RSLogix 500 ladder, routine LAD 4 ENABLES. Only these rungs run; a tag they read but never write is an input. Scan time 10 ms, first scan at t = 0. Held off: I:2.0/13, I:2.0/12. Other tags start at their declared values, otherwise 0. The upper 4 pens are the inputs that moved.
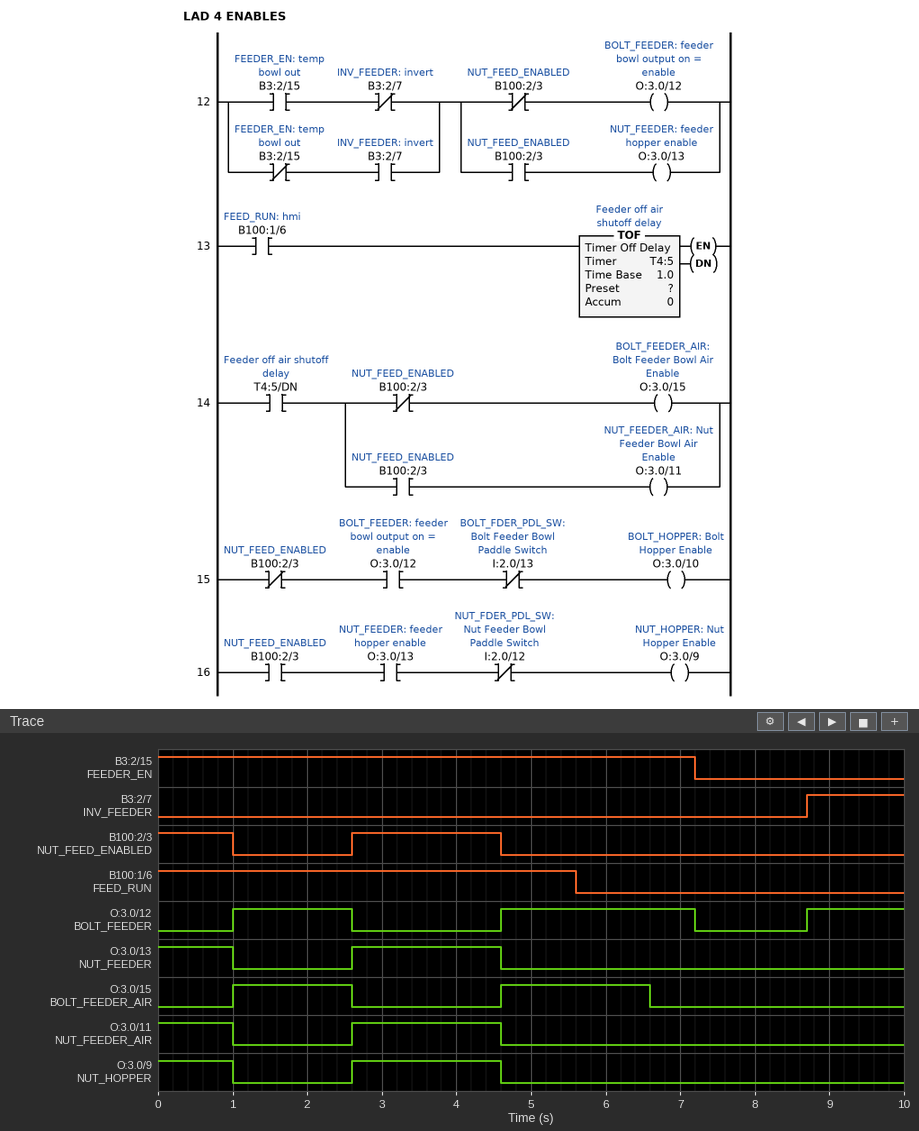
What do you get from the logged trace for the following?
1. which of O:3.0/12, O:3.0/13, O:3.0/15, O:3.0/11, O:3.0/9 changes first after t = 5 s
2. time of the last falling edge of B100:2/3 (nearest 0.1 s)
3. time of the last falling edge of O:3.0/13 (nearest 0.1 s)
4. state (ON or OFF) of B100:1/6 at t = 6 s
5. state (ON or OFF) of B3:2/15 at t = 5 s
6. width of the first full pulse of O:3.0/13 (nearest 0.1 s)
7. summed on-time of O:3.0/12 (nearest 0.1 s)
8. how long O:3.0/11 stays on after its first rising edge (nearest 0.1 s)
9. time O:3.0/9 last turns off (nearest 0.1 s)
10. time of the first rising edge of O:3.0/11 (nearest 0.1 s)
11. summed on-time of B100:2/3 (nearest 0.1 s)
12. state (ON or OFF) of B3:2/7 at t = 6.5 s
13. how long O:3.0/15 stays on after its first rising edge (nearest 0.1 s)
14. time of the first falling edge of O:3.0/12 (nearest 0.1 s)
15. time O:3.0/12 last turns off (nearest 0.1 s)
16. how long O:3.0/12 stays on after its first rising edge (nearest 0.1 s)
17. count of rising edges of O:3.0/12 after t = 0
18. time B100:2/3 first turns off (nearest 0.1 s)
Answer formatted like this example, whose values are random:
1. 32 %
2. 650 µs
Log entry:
1. O:3.0/15
2. 4.6 s
3. 4.6 s
4. OFF
5. ON
6. 2.0 s
7. 5.5 s
8. 2.0 s
9. 4.6 s
10. 2.6 s
11. 3.0 s
12. OFF
13. 1.6 s
14. 2.6 s
15. 7.2 s
16. 1.6 s
17. 3
18. 1.0 s
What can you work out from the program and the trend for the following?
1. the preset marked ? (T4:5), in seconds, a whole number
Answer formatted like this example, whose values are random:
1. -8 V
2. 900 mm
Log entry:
1. 1 s
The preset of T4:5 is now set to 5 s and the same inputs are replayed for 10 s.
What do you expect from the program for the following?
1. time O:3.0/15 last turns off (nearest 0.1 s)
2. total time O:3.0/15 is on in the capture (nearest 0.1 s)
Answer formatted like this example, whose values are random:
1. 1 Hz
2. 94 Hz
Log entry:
1. 2.6 s
2. 7.0 s
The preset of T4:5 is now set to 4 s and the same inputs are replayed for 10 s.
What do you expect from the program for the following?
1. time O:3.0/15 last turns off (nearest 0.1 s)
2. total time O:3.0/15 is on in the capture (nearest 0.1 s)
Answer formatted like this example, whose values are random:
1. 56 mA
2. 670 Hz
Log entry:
1. 9.6 s
2. 6.6 s
